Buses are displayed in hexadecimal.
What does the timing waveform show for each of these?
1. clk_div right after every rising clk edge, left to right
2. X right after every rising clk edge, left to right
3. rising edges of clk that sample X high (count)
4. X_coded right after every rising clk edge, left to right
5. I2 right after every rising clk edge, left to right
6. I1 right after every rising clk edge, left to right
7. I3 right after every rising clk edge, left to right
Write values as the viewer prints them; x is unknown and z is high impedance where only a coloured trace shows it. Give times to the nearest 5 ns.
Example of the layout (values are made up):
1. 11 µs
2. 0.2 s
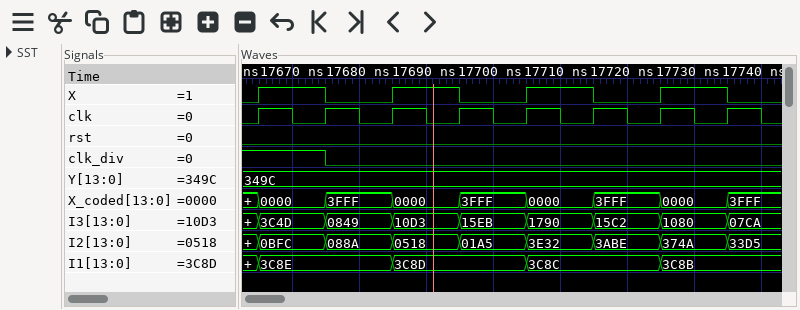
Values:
1. 1 0 0 0 0 0 0 0
2. 1 0 1 0 1 0 1 0
3. 4
4. 0000, 3FFF, 0000, 3FFF, 0000, 3FFF, 0000, 3FFF
5. 0BFC, 088A, 0518, 01A5, 3E32, 3ABE, 374A, 33D5
6. 3C8E, 3C8E, 3C8D, 3C8D, 3C8C, 3C8C, 3C8B, 3C8B
7. 3C4D, 0849, 10D3, 15EB, 1790, 15C2, 1080, 07CA
